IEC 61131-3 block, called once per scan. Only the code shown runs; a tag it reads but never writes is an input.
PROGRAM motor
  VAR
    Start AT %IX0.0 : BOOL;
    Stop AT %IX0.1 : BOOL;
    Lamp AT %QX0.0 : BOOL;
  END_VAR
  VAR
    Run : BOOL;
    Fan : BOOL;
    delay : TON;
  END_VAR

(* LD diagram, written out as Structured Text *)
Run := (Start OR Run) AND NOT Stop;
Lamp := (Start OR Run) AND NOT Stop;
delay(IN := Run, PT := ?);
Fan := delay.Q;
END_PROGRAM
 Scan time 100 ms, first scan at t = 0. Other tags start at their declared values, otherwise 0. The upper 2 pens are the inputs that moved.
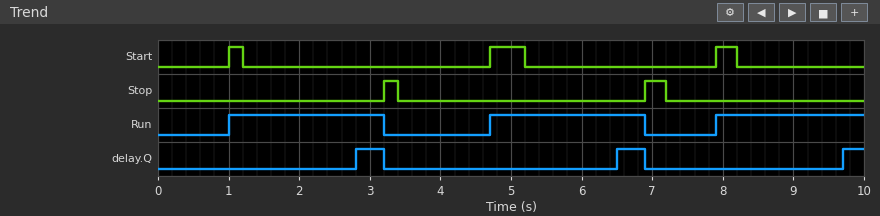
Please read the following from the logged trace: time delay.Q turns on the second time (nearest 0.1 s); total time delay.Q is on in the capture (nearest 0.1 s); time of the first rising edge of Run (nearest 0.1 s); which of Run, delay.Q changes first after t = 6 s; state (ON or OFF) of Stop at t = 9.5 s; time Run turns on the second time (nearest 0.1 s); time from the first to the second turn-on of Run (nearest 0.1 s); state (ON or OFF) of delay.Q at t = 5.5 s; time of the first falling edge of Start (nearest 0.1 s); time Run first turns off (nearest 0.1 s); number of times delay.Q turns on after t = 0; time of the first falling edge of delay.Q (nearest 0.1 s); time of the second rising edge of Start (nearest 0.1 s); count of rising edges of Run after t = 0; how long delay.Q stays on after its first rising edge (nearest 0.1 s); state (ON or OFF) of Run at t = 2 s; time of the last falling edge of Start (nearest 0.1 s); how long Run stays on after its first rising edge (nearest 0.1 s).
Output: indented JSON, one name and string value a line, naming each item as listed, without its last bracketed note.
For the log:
{
  "time delay.Q turns on the second time": "6.5 s",
  "total time delay.Q is on in the capture": "1.1 s",
  "time of the first rising edge of Run": "1.0 s",
  "which of Run, delay.Q changes first after t = 6 s": "delay.Q",
  "state (ON or OFF) of Stop at t = 9.5 s": "OFF",
  "time Run turns on the second time": "4.7 s",
  "time from the first to the second turn-on of Run": "3.7 s",
  "state (ON or OFF) of delay.Q at t = 5.5 s": "OFF",
  "time of the first falling edge of Start": "1.2 s",
  "time Run first turns off": "3.2 s",
  "number of times delay.Q turns on after t = 0": "3",
  "time of the first falling edge of delay.Q": "3.2 s",
  "time of the second rising edge of Start": "4.7 s",
  "count of rising edges of Run after t = 0": "3",
  "how long delay.Q stays on after its first rising edge": "0.4 s",
  "state (ON or OFF) of Run at t = 2 s": "ON",
  "time of the last falling edge of Start": "8.2 s",
  "how long Run stays on after its first rising edge": "2.2 s"
}
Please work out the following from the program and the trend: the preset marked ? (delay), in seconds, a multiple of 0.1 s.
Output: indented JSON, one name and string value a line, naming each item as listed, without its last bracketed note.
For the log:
{
  "the preset marked ? (delay), in seconds, a multiple of 0.1 s": "1.8 s"
}
